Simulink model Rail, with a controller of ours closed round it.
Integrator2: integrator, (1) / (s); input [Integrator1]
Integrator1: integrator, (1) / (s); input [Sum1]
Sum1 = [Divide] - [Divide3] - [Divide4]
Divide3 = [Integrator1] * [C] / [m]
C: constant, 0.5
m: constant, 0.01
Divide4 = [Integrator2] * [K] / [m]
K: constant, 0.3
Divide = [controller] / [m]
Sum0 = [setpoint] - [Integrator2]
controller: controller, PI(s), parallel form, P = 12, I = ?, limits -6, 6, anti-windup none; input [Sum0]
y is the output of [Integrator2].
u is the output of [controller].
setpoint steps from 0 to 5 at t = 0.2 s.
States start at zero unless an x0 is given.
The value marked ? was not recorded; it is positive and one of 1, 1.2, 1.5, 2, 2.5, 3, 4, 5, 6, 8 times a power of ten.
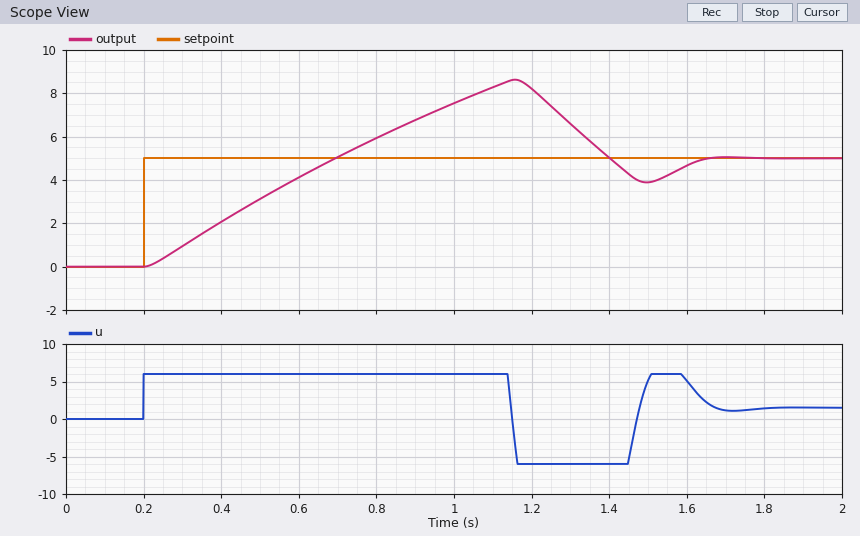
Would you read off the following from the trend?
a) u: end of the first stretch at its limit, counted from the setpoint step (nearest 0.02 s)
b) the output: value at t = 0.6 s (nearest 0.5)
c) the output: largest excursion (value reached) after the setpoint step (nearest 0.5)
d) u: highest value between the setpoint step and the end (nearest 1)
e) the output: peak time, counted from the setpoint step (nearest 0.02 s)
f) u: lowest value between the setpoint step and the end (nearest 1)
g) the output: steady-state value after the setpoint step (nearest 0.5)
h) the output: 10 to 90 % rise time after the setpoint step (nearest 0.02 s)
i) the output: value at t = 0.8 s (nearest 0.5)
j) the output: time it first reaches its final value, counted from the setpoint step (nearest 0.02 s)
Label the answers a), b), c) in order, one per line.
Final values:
a) 0.94 s
b) 4.0
c) 8.5
d) 6
e) 0.96 s
f) -6
g) 5.0
h) 0.38 s
i) 6.0
j) 0.50 s
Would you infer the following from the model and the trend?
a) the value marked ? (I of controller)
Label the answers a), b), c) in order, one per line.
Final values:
a) 120
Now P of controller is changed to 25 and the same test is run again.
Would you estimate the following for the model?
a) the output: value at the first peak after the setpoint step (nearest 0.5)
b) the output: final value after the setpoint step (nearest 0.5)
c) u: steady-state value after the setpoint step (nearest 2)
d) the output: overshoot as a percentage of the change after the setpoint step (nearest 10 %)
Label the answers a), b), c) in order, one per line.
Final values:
a) 8.0
b) 5.0
c) 2
d) 60 %
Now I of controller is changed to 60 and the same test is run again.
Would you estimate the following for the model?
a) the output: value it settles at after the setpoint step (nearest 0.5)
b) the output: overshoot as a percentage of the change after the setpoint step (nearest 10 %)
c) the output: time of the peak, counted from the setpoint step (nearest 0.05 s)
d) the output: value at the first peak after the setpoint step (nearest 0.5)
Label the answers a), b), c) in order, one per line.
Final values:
a) 5.0
b) 60 %
c) 0.90 s
d) 8.0
